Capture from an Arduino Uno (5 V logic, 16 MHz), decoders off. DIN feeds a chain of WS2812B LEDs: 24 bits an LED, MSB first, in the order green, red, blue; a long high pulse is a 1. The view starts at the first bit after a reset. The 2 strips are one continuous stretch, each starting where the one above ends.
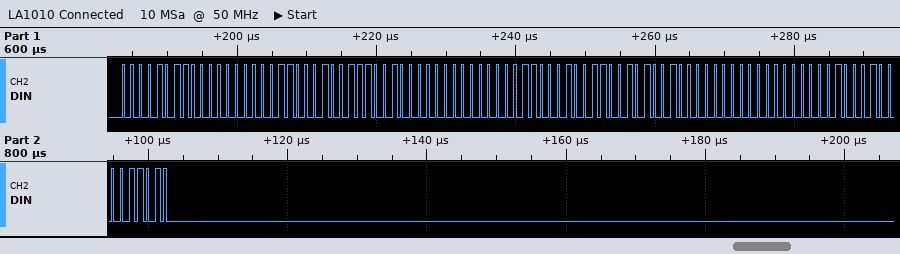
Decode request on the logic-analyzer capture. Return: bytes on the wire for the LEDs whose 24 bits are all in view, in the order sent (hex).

0B 00 31 39 00 03 13 29 00 00 22 1A
